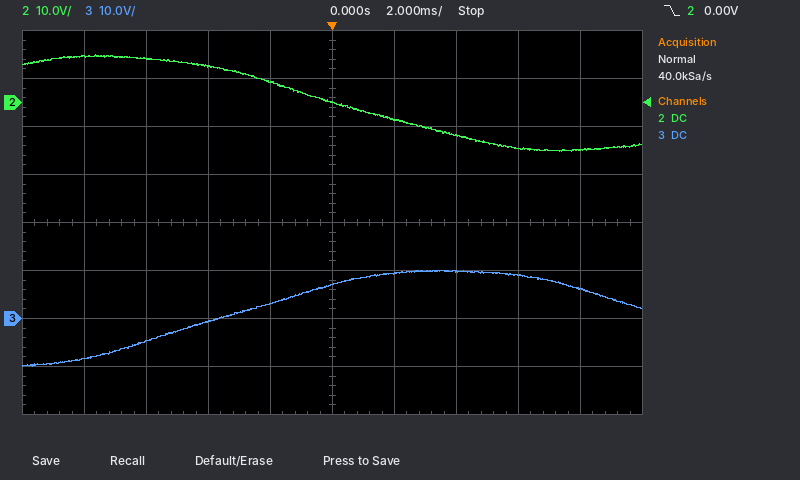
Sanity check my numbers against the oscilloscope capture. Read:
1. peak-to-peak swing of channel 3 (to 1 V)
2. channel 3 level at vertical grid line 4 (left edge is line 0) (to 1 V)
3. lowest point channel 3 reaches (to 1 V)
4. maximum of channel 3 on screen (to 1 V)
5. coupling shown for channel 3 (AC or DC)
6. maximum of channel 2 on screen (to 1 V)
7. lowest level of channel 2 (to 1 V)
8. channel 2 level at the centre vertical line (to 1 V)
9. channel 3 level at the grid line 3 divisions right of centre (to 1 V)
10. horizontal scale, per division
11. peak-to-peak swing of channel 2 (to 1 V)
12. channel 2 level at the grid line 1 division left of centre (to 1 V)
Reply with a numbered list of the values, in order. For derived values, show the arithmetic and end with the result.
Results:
1. 10 V − (-10 V) = 20 V
2. 3 V
3. -10 V
4. 10 V
5. DC
6. 10 V
7. -10 V
8. 0 V
9. 9 V
10. 2 ms
11. 10 V − (-10 V) = 20 V
12. 4 V
